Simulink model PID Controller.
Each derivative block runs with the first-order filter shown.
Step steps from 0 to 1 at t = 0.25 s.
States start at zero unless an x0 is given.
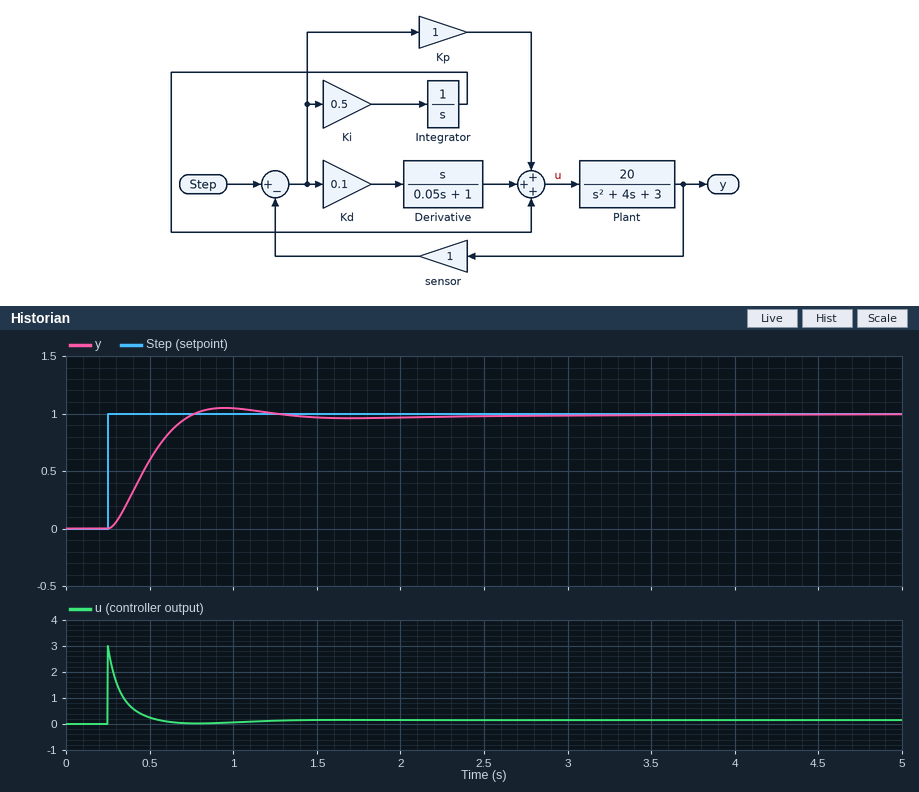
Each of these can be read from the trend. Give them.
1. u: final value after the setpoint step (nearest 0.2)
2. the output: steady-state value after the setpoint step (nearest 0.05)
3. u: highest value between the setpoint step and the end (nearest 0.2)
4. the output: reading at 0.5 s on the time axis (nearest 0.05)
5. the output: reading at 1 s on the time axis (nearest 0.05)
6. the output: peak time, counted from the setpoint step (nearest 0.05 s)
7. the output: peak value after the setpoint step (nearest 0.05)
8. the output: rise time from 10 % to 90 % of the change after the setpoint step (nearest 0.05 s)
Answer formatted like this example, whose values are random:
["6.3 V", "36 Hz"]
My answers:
["0.2", "1.00", "3.0", "0.60", "1.05", "0.70 s", "1.05", "0.35 s"]
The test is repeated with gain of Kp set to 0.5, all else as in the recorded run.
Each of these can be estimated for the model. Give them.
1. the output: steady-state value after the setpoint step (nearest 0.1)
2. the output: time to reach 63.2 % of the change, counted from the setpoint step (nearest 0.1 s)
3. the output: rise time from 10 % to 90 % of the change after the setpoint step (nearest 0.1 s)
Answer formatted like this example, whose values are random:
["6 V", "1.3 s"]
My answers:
["1.0", "0.4 s", "0.6 s"]
